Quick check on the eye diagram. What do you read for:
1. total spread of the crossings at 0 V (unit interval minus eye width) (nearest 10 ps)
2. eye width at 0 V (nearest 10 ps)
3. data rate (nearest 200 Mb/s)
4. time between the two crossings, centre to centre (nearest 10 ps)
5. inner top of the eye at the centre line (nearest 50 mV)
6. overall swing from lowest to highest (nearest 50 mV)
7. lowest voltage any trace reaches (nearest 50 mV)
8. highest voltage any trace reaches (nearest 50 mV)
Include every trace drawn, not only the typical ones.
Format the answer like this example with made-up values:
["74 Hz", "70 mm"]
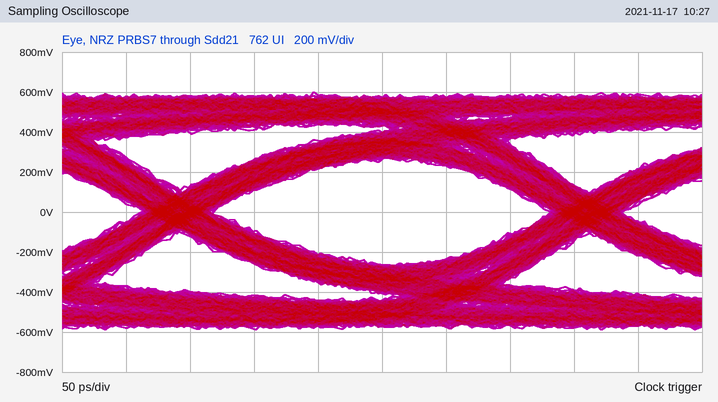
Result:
["60 ps", "260 ps", "3.2 Gb/s", "320 ps", "250 mV", "1.20 V", "-600 mV", "600 mV"]
